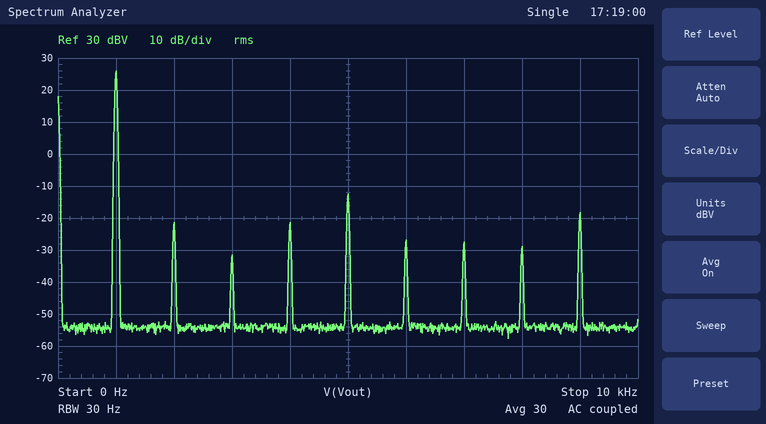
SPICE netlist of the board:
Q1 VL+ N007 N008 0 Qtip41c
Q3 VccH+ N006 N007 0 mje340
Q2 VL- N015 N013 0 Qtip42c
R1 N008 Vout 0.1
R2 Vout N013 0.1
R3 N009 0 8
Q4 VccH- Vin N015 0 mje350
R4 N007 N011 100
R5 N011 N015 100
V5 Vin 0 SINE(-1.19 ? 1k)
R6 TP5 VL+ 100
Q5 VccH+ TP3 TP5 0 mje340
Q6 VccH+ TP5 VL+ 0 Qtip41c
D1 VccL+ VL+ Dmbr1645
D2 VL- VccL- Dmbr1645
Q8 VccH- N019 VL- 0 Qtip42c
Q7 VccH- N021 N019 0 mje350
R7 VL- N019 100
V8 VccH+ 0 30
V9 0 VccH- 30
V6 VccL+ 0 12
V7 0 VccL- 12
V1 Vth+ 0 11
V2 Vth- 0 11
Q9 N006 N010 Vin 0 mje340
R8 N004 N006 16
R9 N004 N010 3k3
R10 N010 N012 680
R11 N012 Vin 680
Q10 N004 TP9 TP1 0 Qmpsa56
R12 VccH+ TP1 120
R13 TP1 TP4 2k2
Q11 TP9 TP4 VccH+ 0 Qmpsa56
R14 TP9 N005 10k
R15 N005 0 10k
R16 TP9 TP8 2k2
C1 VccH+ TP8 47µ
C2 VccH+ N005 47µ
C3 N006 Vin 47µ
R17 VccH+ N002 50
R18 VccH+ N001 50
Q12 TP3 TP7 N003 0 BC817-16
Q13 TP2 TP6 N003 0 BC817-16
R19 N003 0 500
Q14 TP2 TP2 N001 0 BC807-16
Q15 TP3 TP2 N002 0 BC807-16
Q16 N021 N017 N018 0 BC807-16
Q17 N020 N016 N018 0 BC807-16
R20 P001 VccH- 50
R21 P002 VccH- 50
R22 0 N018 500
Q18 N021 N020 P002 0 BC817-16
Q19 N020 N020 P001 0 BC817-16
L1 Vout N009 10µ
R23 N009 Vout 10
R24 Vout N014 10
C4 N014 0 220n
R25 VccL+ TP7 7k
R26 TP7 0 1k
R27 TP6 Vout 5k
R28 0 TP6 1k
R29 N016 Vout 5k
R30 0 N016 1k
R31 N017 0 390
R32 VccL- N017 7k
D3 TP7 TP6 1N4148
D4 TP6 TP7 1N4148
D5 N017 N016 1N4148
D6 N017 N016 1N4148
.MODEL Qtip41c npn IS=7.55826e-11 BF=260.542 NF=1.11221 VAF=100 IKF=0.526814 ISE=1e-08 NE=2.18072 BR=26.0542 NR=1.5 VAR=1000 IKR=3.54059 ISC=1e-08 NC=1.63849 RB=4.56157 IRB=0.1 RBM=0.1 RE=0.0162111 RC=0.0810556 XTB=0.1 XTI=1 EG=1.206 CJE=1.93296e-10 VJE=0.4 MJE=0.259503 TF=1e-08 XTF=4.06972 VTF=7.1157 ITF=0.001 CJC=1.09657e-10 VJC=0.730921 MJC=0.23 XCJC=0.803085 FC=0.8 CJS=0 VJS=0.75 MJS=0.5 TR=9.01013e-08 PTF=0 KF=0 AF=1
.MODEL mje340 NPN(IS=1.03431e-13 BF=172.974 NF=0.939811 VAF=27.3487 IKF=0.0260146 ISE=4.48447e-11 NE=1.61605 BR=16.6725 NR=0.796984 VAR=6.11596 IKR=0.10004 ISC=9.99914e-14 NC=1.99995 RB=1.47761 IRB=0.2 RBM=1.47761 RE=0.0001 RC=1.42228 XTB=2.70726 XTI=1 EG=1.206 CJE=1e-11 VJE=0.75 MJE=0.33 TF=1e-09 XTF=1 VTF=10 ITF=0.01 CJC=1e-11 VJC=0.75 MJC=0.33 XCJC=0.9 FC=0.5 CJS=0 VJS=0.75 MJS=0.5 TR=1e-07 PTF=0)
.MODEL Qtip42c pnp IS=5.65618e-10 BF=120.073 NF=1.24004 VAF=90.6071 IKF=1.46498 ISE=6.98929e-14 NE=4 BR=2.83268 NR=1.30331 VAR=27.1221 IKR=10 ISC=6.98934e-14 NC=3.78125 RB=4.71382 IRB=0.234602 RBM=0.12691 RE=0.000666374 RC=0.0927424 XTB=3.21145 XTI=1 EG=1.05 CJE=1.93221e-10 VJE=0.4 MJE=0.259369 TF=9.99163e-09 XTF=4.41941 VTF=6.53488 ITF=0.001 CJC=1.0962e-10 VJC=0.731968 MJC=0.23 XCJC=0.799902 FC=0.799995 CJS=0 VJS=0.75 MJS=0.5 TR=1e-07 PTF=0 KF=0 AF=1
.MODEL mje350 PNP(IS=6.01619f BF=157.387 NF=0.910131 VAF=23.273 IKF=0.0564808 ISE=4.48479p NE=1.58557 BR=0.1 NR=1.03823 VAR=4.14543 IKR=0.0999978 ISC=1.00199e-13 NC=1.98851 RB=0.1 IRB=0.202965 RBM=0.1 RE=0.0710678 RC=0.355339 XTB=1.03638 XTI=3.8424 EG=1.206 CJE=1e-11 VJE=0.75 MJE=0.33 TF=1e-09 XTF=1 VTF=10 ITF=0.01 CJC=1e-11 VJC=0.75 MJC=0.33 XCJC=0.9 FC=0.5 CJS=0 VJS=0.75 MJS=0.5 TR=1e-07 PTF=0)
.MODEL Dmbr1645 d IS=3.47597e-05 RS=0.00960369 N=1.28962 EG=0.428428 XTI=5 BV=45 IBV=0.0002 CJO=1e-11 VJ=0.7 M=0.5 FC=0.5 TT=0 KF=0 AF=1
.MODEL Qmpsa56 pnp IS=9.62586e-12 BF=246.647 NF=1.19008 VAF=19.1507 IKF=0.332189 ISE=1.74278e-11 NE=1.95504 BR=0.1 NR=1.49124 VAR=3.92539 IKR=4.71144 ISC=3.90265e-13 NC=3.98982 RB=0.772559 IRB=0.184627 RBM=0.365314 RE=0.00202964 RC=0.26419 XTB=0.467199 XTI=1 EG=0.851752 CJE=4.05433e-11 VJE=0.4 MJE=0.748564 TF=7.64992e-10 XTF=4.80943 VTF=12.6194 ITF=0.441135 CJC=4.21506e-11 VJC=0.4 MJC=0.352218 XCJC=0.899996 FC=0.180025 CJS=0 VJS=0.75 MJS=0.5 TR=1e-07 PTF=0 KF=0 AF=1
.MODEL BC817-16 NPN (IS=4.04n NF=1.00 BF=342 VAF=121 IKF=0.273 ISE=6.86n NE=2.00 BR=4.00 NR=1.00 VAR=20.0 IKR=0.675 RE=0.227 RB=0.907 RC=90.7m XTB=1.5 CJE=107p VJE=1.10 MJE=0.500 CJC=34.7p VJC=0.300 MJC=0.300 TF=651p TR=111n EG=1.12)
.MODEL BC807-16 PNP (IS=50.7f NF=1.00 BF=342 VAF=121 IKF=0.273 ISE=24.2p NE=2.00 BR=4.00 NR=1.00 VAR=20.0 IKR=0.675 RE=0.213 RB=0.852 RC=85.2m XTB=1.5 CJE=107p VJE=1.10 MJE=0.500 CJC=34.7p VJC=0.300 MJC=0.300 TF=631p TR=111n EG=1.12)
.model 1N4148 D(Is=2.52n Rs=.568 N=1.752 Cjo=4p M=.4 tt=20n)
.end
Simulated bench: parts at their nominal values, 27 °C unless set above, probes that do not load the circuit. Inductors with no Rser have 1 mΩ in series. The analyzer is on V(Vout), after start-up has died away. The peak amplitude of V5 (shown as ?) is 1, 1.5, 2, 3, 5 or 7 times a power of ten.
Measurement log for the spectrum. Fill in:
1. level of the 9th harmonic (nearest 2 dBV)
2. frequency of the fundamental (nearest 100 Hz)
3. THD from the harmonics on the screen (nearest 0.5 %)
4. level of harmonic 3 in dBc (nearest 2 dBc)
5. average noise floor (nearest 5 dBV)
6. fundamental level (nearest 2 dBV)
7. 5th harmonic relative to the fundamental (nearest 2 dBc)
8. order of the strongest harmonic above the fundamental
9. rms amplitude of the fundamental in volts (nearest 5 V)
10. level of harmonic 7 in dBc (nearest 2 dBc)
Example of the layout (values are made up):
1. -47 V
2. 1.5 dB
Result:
1. -18 dBV
2. 1.0 kHz
3. 1.5 %
4. -58 dBc
5. -55 dBV
6. 26 dBV
7. -38 dBc
8. 5
9. 20 V
10. -54 dBc
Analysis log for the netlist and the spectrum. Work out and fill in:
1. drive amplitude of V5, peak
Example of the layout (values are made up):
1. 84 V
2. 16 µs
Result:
1. 30 V
